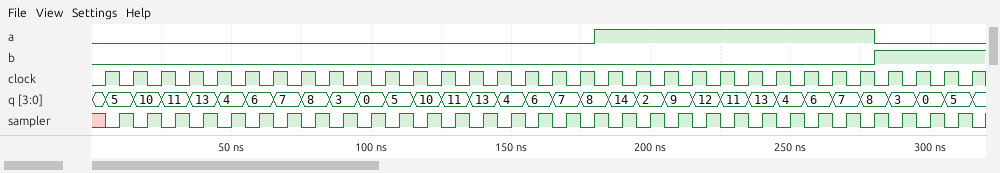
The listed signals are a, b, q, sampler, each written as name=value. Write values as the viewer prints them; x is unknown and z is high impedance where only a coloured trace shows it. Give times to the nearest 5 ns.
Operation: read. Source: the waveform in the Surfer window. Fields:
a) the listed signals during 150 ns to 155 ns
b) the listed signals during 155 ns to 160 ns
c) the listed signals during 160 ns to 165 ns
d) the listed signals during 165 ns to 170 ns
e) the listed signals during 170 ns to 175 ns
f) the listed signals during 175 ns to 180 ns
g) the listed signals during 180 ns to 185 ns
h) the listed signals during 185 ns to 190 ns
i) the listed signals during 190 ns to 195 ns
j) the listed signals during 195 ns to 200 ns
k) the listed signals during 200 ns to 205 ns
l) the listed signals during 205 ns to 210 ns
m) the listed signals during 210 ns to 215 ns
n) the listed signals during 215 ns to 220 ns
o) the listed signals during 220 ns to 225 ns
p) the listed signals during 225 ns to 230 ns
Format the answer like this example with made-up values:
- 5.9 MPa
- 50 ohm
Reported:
- a=0, b=0, q=4, sampler=1
- a=0, b=0, q=6, sampler=0
- a=0, b=0, q=6, sampler=1
- a=0, b=0, q=7, sampler=0
- a=0, b=0, q=7, sampler=1
- a=0, b=0, q=8, sampler=0
- a=1, b=0, q=8, sampler=1
- a=1, b=0, q=14, sampler=0
- a=1, b=0, q=14, sampler=1
- a=1, b=0, q=2, sampler=0
- a=1, b=0, q=2, sampler=1
- a=1, b=0, q=9, sampler=0
- a=1, b=0, q=9, sampler=1
- a=1, b=0, q=12, sampler=0
- a=1, b=0, q=12, sampler=1
- a=1, b=0, q=11, sampler=0
